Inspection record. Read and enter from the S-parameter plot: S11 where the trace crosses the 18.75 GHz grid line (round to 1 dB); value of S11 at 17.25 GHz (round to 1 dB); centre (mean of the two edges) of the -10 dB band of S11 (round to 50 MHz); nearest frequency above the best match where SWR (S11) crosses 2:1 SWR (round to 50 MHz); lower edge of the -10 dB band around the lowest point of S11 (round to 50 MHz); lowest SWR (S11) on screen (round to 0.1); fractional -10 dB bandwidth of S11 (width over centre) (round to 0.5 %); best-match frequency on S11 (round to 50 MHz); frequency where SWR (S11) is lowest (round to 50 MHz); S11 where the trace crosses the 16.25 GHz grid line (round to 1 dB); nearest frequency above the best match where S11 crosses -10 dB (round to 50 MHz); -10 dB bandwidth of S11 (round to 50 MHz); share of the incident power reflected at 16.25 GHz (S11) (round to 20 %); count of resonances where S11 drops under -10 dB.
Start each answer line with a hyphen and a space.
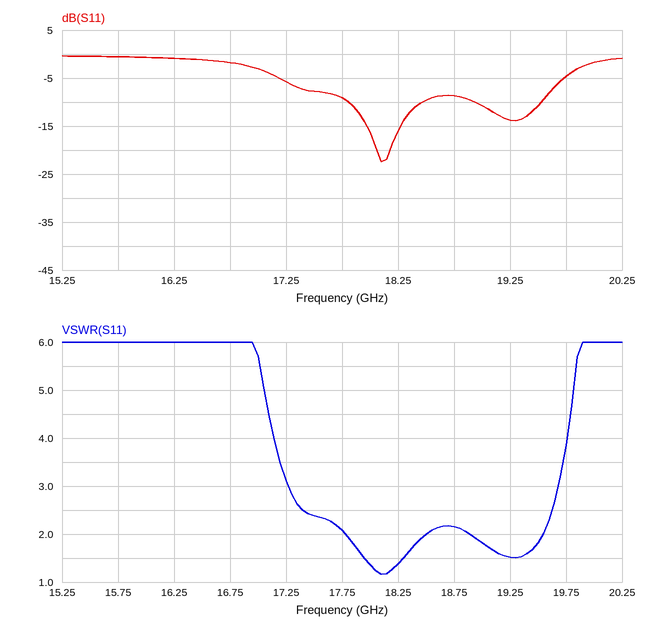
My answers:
- -9 dB
- -6 dB
- 18.15 GHz
- 18.50 GHz
- 17.80 GHz
- 1.2
- 3.5 %
- 18.10 GHz
- 18.10 GHz
- -1 dB
- 18.45 GHz
- 650 MHz
- 80 %
- 2
